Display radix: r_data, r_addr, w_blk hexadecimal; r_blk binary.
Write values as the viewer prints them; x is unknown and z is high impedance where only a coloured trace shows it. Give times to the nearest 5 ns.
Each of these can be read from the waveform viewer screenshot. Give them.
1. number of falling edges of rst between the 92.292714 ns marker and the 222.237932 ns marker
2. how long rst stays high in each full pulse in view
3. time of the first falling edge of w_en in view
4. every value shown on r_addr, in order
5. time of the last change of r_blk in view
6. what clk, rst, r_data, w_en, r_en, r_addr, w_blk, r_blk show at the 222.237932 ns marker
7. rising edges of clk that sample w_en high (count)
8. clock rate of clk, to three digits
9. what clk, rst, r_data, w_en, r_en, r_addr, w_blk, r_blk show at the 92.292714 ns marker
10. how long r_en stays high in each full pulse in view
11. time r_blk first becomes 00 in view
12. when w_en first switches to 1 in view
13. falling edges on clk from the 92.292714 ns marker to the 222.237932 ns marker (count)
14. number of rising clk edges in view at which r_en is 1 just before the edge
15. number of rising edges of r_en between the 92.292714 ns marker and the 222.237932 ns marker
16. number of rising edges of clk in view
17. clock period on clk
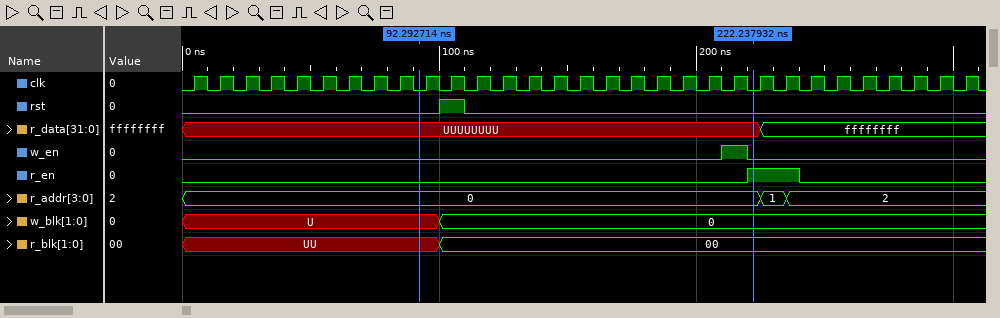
1
10 ns
220 ns
0, 1, 2
100 ns
clk=0, rst=0, r_data=UUUUUUUU, w_en=0, r_en=1, r_addr=0, w_blk=0, r_blk=00
1
100 MHz
clk=0, rst=0, r_data=UUUUUUUU, w_en=0, r_en=0, r_addr=0, w_blk=U, r_blk=UU
20 ns
100 ns
210 ns
13
2
1
31
10 ns
